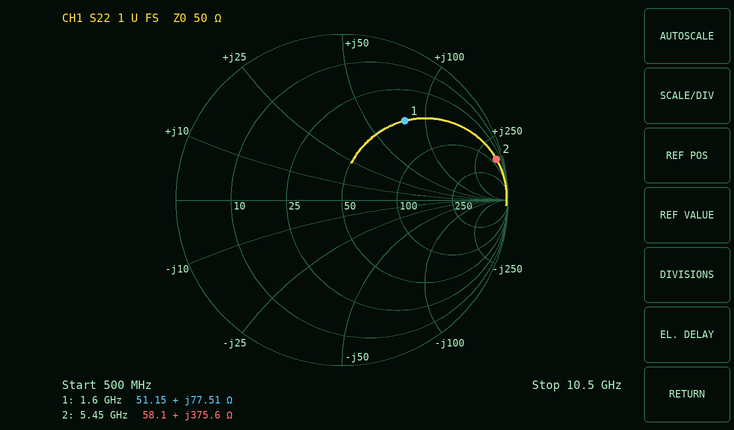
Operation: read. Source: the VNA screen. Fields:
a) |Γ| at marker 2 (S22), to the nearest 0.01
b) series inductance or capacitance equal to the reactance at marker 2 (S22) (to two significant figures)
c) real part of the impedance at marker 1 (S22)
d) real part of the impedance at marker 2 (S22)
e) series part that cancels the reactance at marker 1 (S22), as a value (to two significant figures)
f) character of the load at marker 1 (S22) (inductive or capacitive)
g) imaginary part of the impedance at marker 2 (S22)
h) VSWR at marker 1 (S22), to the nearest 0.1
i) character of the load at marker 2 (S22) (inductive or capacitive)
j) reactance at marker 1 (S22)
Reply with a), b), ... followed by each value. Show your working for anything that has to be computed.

a) 0.96
b) L = 375.6 Ω/(2π × 5.45 GHz) ≈ 11 nH
c) 51.15 Ω
d) 58.1 Ω
e) C = 1/(2π × 1.6 GHz × 77.51 Ω) ≈ 1.3 pF
f) inductive
g) +375.6 Ω
h) 4.1
i) inductive
j) +77.51 Ω
